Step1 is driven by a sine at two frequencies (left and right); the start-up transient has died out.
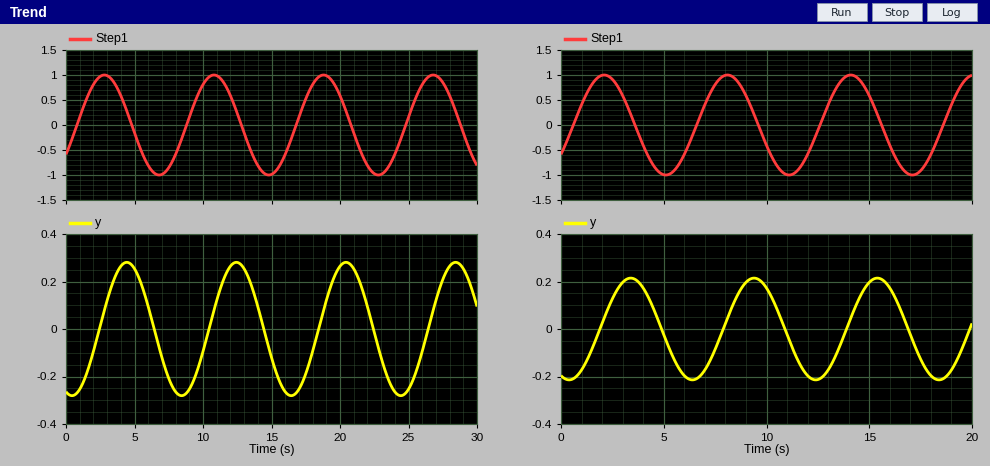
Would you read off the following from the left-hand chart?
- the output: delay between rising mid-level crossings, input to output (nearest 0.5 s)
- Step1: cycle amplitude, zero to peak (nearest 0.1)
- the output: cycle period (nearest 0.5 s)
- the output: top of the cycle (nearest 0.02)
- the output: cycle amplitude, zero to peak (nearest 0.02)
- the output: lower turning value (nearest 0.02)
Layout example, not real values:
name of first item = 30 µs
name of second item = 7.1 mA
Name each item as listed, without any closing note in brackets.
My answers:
the output: delay between rising mid-level crossings, input to output = 1.5 s
Step1: cycle amplitude, zero to peak = 1.0
the output: cycle period = 8.0 s
the output: top of the cycle = 0.28
the output: cycle amplitude, zero to peak = 0.28
the output: lower turning value = -0.28
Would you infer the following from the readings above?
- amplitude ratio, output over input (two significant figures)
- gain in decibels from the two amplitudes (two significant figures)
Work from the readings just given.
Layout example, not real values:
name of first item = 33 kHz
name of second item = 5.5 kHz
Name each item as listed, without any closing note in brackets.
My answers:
amplitude ratio, output over input = 0.28
gain in decibels from the two amplitudes = -11 dB
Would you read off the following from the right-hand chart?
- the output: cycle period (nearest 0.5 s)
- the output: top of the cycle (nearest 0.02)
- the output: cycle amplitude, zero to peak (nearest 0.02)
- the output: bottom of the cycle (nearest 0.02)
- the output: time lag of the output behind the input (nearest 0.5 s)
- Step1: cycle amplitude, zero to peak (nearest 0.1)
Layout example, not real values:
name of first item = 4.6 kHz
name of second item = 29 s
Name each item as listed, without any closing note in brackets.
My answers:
the output: cycle period = 6.0 s
the output: top of the cycle = 0.22
the output: cycle amplitude, zero to peak = 0.22
the output: bottom of the cycle = -0.22
the output: time lag of the output behind the input = 1.5 s
Step1: cycle amplitude, zero to peak = 1.0
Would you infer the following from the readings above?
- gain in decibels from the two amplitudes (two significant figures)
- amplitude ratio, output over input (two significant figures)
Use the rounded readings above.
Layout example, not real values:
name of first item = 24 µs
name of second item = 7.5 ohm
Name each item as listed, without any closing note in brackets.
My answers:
gain in decibels from the two amplitudes = -13 dB
amplitude ratio, output over input = 0.22
